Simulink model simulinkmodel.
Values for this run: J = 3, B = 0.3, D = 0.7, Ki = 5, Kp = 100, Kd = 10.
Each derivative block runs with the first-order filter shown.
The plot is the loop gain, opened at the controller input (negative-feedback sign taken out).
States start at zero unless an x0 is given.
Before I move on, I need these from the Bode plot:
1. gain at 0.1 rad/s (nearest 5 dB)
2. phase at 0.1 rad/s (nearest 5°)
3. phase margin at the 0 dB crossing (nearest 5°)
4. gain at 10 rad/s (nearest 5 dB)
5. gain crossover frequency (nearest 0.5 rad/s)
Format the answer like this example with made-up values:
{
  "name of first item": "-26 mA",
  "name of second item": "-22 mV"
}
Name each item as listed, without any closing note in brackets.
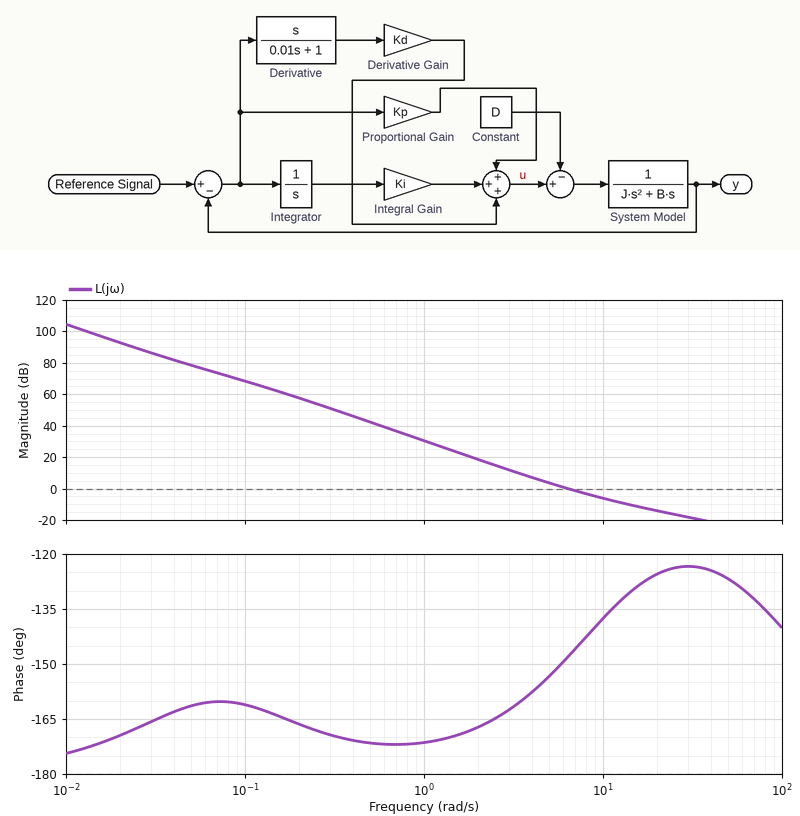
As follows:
{
  "gain at 0.1 rad/s": "70 dB",
  "phase at 0.1 rad/s": "-160°",
  "phase margin at the 0 dB crossing": "30°",
  "gain at 10 rad/s": "-5 dB",
  "gain crossover frequency": "6.5 rad/s"
}
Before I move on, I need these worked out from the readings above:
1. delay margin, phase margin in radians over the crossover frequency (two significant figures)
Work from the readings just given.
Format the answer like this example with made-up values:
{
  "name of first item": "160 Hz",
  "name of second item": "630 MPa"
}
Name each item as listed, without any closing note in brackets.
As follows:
{
  "delay margin, phase margin in radians over the crossover frequency": "0.081 s"
}
